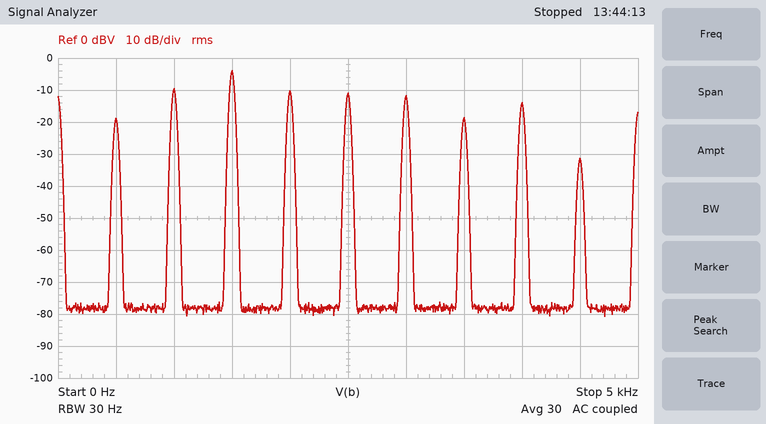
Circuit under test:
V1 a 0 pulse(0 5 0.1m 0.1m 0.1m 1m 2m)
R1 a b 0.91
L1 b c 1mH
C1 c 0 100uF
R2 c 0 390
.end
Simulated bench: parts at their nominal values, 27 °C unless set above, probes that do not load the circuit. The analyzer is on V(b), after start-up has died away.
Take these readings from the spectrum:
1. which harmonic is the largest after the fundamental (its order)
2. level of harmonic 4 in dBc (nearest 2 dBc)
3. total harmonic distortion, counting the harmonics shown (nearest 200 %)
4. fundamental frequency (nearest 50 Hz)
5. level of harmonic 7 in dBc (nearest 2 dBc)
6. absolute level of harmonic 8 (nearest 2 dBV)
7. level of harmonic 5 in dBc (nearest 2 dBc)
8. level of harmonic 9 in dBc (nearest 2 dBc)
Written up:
3
8 dBc
800 %
500 Hz
0 dBc
-14 dBV
8 dBc
-12 dBc
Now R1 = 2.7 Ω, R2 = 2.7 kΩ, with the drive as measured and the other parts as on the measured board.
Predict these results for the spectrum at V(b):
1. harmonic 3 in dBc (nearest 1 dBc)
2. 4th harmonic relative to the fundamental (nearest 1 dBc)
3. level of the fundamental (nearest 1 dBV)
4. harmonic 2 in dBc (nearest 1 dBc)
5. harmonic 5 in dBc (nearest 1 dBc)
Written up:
25 dBc
19 dBc
-29 dBV
19 dBc
18 dBc
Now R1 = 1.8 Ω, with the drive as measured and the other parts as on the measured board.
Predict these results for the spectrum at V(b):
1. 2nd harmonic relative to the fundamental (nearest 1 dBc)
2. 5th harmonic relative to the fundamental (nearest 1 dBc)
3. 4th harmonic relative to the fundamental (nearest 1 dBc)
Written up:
15 dBc
14 dBc
14 dBc
